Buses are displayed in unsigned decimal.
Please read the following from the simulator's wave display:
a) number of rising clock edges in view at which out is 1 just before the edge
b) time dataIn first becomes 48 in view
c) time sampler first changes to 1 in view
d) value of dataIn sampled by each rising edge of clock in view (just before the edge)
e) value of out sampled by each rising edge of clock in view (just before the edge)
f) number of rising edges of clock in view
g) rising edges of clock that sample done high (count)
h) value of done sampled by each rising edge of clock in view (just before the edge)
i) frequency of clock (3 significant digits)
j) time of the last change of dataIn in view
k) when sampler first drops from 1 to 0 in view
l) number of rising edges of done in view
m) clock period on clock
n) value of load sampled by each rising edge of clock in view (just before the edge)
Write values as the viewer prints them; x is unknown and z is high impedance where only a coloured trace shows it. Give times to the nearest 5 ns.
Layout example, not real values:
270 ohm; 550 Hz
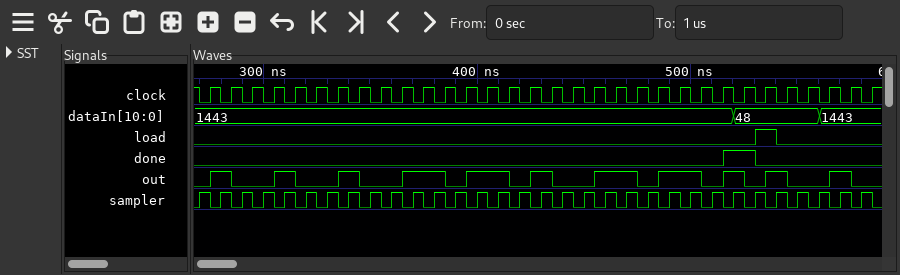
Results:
15; 520 ns; 270 ns; 1443, 1443, 1443, 1443, 1443, 1443, 1443, 1443, 1443, 1443, 1443, 1443, 1443, 1443, 1443, 1443, 1443, 1443, 1443, 1443, 1443, 1443, 1443, 1443, 1443, 48, 48, 48, 48, 1443, 1443, 1443; 0 1 0 0 1 0 0 1 0 0 1 1 0 1 1 0 1 0 0 1 1 0 1 1 0 1 0 1 0 0 1 0; 32; 1; 0 0 0 0 0 0 0 0 0 0 0 0 0 0 0 0 0 0 0 0 0 0 0 0 0 1 0 0 0 0 0 0; 100 MHz; 560 ns; 275 ns; 1; 10 ns; 0 0 0 0 0 0 0 0 0 0 0 0 0 0 0 0 0 0 0 0 0 0 0 0 0 0 1 0 0 0 0 0
